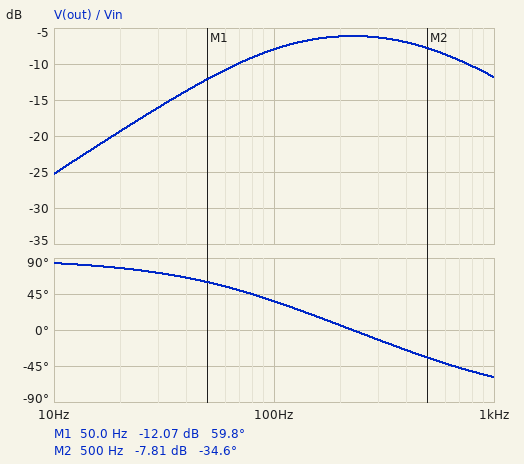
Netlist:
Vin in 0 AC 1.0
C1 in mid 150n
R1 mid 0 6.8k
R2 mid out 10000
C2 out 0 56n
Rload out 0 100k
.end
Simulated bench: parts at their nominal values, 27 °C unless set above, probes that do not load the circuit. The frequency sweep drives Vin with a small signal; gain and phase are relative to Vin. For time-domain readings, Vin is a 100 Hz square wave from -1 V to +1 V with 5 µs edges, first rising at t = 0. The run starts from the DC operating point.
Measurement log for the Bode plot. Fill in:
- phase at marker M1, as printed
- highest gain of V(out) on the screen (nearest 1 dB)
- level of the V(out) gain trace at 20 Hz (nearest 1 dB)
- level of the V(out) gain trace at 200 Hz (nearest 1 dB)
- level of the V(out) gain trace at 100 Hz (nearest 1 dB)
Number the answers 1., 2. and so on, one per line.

1. 59.8 deg
2. -6 dB
3. -19 dB
4. -6 dB
5. -8 dB
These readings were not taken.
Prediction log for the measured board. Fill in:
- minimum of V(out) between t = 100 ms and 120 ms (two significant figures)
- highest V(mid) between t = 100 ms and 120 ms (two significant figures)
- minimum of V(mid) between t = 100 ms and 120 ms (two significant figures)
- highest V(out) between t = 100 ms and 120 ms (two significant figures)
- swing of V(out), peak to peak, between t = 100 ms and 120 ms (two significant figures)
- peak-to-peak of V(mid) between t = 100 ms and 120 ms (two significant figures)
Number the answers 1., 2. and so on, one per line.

1. -750 mV
2. 2.0 V
3. -2.0 V
4. 750 mV
5. 1.5 V
6. 3.9 V
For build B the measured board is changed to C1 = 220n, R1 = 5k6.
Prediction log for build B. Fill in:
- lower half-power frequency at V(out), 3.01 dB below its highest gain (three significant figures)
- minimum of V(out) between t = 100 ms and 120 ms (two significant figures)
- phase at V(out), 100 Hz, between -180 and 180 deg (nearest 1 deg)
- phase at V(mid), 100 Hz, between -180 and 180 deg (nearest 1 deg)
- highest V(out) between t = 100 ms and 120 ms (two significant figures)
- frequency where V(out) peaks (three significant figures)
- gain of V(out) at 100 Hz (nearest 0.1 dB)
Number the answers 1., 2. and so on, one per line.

1. 72.4 Hz
2. -830 mV
3. 32 deg
4. 50 deg
5. 830 mV
6. 206 Hz
7. -6.6 dB
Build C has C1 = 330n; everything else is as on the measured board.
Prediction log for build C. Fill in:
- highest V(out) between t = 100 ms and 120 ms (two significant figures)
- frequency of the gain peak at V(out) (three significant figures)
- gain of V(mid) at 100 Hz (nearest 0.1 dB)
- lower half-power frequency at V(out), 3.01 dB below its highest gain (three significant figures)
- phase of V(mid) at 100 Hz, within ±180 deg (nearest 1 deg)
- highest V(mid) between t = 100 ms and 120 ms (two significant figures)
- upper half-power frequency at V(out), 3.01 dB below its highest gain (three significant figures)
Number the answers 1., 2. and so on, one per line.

1. 920 mV
2. 153 Hz
3. -2.8 dB
4. 49.0 Hz
5. 35 deg
6. 1.8 V
7. 481 Hz
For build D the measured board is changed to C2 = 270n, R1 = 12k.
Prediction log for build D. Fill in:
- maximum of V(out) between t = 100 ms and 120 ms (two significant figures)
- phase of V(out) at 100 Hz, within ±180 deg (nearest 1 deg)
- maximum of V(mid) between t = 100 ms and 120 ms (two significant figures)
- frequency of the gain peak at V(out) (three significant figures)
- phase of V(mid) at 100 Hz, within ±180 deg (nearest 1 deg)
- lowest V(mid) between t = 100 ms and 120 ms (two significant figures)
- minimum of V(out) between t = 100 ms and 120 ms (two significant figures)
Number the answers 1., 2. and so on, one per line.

1. 260 mV
2. -8 deg
3. 1.9 V
4. 79.7 Hz
5. 49 deg
6. -1.9 V
7. -260 mV
